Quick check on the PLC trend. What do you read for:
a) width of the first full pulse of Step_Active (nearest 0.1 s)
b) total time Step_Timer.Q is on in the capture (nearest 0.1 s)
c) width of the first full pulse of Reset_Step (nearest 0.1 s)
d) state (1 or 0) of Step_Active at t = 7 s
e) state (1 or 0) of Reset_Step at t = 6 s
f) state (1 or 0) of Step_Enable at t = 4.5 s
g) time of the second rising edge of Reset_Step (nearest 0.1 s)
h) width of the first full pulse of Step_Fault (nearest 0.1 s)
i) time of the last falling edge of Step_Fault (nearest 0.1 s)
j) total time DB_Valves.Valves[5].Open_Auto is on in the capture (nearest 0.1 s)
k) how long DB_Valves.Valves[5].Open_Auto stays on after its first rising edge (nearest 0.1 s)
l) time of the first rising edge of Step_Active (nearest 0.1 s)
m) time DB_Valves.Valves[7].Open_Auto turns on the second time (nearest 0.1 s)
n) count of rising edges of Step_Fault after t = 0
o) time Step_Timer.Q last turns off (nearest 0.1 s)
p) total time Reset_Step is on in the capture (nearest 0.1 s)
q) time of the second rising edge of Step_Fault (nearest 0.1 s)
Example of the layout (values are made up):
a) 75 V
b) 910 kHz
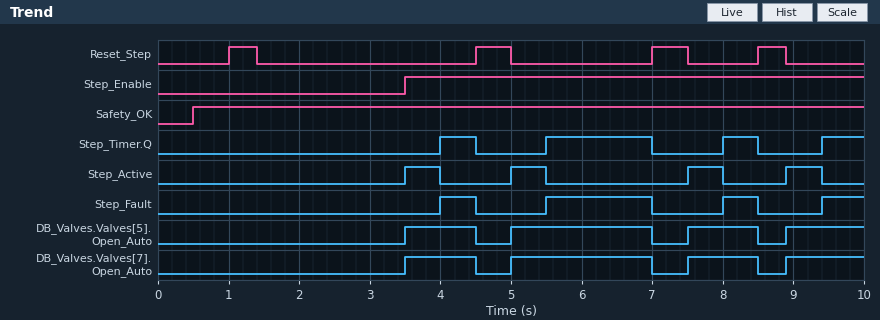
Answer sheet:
a) 0.5 s
b) 3.1 s
c) 0.4 s
d) 0
e) 0
f) 1
g) 4.5 s
h) 0.5 s
i) 8.5 s
j) 5.1 s
k) 1.0 s
l) 3.5 s
m) 5.0 s
n) 4
o) 8.5 s
p) 1.8 s
q) 5.5 s
